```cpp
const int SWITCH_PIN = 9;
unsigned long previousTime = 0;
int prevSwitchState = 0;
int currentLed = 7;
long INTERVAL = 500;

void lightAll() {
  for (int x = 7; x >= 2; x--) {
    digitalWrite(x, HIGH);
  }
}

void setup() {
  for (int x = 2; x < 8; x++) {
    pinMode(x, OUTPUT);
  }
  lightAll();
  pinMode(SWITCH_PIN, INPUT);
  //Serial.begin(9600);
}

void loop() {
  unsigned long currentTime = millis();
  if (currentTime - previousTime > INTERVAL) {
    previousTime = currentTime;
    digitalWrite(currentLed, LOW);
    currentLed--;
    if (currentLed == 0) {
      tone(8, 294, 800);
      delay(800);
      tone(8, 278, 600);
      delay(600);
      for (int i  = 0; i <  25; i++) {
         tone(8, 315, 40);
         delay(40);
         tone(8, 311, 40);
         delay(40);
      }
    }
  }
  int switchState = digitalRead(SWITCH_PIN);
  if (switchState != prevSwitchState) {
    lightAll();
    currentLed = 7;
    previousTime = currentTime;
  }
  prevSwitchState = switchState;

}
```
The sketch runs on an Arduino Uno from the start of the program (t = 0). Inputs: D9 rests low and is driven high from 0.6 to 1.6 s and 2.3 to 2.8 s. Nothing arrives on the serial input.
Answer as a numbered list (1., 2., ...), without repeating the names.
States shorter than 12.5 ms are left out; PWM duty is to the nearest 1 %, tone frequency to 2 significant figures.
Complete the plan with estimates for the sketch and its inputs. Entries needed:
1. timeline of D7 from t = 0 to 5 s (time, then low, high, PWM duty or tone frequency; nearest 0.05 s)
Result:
1. 0 s high; 0.5 s low; 0.6 s high; 1.1 s low; 1.6 s high; 2.1 s low; 2.3 s high; 3.3 s low
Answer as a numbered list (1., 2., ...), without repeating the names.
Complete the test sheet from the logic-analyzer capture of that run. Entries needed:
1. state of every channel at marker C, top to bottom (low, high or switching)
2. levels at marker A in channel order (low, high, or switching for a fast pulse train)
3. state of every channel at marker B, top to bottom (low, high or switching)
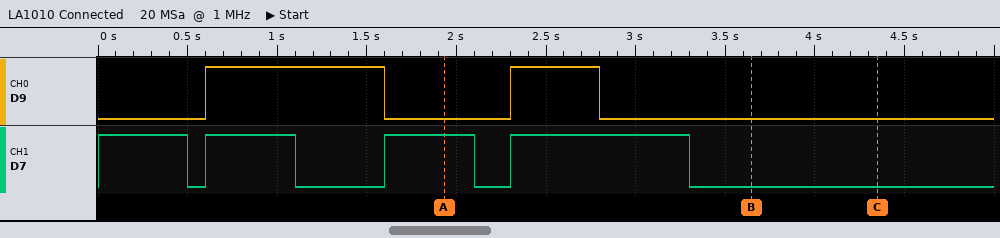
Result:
1. D9 low, D7 low
2. D9 low, D7 high
3. D9 low, D7 low
